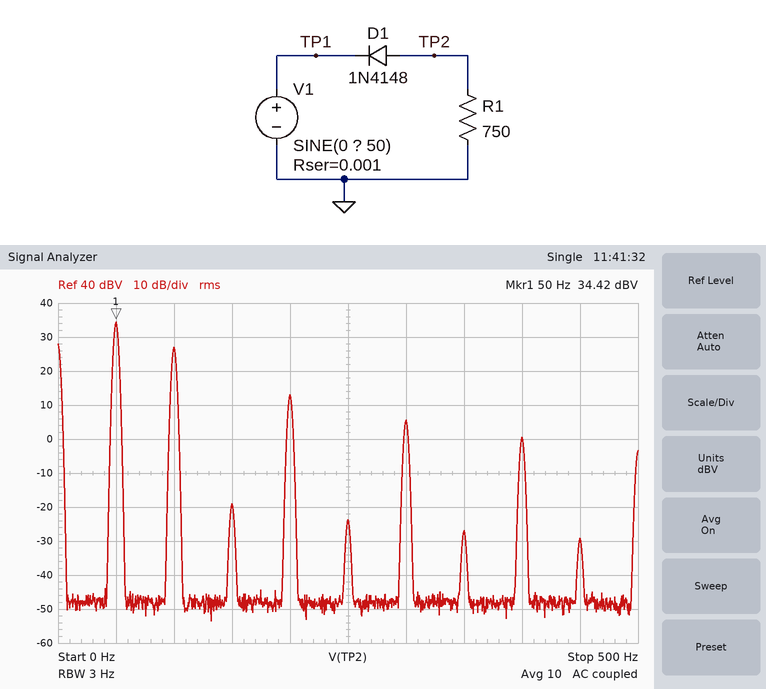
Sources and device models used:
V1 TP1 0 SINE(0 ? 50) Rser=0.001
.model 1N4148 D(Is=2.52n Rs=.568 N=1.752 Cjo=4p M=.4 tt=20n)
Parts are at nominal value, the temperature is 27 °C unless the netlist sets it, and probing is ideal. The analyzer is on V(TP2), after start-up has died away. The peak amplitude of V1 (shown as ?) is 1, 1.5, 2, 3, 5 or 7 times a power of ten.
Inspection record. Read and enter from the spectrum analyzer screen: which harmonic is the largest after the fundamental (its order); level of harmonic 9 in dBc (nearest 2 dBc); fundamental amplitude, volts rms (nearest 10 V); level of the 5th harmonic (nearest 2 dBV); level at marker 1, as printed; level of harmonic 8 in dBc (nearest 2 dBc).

2
-64 dBc
50 V
-24 dBV
34.42 dBV
-34 dBc
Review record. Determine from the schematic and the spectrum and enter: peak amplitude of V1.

150 V
